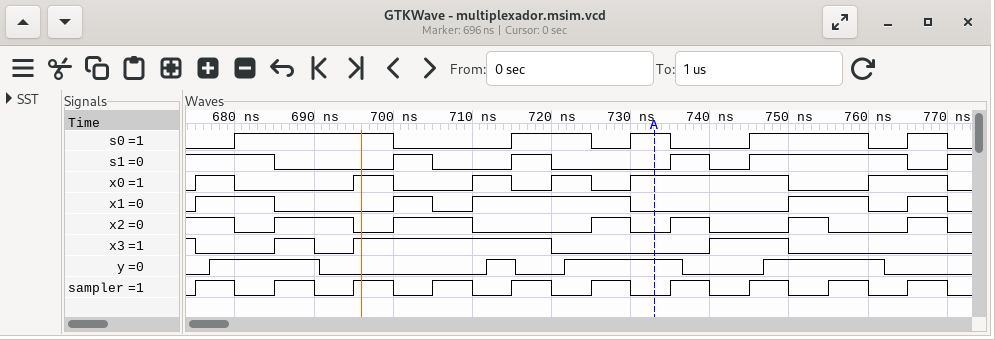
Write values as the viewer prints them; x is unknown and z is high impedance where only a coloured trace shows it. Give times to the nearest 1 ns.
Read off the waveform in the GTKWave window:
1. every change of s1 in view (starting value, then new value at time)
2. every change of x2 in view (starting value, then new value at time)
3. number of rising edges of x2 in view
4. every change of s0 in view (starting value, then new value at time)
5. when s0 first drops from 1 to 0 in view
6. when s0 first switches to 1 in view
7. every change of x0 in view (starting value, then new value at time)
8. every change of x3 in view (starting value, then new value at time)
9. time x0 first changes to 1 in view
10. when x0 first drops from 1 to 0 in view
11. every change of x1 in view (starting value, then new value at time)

1, 0 at 685 ns, 1 at 700 ns, 0 at 705 ns, 1 at 715 ns, 0 at 720 ns, 1 at 735 ns, 0 at 740 ns, 1 at 745 ns, 0 at 765 ns, 1 at 770 ns
1, 0 at 680 ns, 1 at 685 ns, 0 at 695 ns, 1 at 700 ns, 0 at 710 ns, 1 at 725 ns, 0 at 730 ns, 1 at 735 ns, 0 at 740 ns, 1 at 750 ns, 0 at 755 ns, 1 at 765 ns, 0 at 770 ns
6
0, 1 at 680 ns, 0 at 700 ns, 1 at 715 ns, 0 at 725 ns, 1 at 730 ns, 0 at 735 ns, 1 at 745 ns, 0 at 760 ns, 1 at 765 ns, 0 at 770 ns
700 ns
680 ns
0, 1 at 675 ns, 0 at 680 ns, 1 at 695 ns, 0 at 700 ns, 1 at 710 ns, 0 at 715 ns, 1 at 720 ns, 0 at 725 ns, 1 at 730 ns, 0 at 750 ns, 1 at 760 ns, 0 at 770 ns
1, 0 at 675 ns, 1 at 685 ns, 0 at 690 ns, 1 at 695 ns, 0 at 720 ns, 1 at 740 ns, 0 at 750 ns
675 ns
680 ns
0, 1 at 675 ns, 0 at 685 ns, 1 at 700 ns, 0 at 705 ns, 1 at 710 ns, 0 at 730 ns, 1 at 750 ns, 0 at 760 ns, 1 at 765 ns, 0 at 770 ns
